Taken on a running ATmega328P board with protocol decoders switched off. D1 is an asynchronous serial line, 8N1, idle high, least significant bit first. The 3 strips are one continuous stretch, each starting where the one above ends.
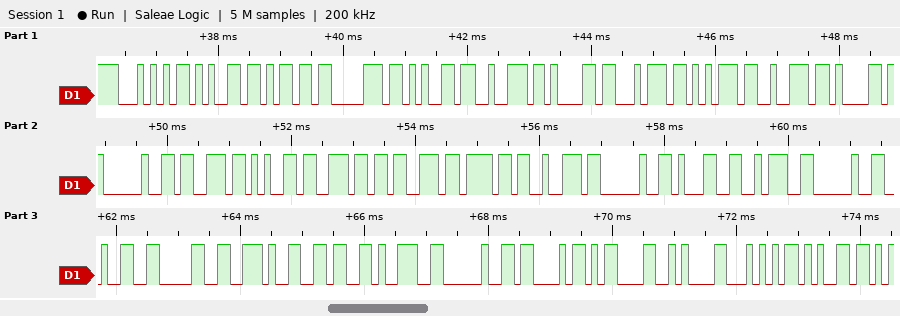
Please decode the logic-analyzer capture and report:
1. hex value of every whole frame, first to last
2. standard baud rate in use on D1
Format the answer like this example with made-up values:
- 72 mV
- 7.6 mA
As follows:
- 54 65 6D 70 65 72 61 74 75 72 61 20 73 65 6E 73 6F 72 20 31 3A 20 32 30 2E 36 39 20 43 0D 0A 54 65
- 9600 baud
